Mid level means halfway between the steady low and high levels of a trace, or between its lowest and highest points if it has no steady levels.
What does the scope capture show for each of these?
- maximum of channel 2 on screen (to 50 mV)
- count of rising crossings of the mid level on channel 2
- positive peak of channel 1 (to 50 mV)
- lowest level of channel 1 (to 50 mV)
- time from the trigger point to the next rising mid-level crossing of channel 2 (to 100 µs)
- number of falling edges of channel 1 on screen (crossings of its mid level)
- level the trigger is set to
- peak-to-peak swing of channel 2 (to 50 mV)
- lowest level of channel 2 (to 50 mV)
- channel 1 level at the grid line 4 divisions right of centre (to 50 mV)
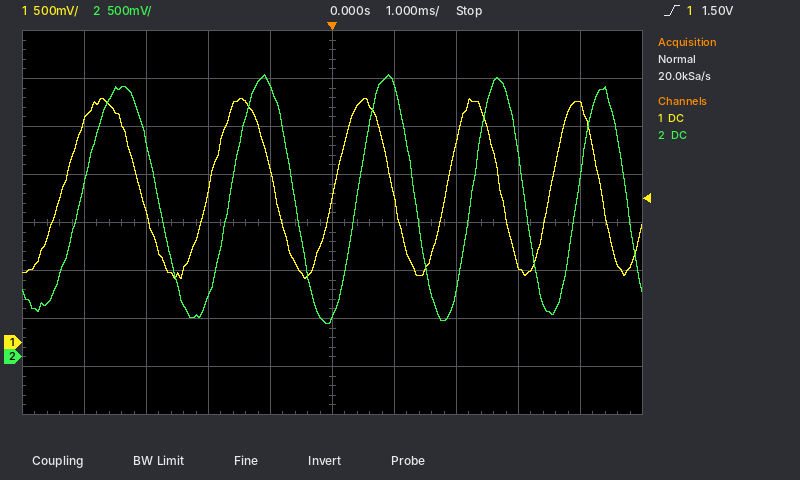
2.95 V
5
2.55 V
650 mV
400 µs
5
1.50 V
2.60 V
350 mV
2.45 V
